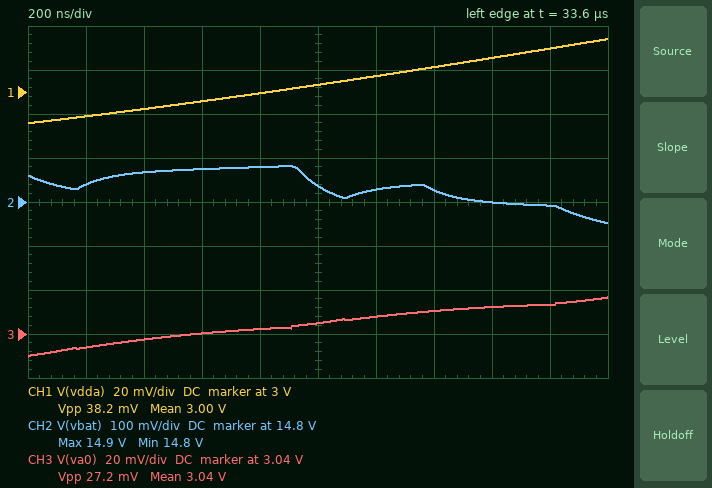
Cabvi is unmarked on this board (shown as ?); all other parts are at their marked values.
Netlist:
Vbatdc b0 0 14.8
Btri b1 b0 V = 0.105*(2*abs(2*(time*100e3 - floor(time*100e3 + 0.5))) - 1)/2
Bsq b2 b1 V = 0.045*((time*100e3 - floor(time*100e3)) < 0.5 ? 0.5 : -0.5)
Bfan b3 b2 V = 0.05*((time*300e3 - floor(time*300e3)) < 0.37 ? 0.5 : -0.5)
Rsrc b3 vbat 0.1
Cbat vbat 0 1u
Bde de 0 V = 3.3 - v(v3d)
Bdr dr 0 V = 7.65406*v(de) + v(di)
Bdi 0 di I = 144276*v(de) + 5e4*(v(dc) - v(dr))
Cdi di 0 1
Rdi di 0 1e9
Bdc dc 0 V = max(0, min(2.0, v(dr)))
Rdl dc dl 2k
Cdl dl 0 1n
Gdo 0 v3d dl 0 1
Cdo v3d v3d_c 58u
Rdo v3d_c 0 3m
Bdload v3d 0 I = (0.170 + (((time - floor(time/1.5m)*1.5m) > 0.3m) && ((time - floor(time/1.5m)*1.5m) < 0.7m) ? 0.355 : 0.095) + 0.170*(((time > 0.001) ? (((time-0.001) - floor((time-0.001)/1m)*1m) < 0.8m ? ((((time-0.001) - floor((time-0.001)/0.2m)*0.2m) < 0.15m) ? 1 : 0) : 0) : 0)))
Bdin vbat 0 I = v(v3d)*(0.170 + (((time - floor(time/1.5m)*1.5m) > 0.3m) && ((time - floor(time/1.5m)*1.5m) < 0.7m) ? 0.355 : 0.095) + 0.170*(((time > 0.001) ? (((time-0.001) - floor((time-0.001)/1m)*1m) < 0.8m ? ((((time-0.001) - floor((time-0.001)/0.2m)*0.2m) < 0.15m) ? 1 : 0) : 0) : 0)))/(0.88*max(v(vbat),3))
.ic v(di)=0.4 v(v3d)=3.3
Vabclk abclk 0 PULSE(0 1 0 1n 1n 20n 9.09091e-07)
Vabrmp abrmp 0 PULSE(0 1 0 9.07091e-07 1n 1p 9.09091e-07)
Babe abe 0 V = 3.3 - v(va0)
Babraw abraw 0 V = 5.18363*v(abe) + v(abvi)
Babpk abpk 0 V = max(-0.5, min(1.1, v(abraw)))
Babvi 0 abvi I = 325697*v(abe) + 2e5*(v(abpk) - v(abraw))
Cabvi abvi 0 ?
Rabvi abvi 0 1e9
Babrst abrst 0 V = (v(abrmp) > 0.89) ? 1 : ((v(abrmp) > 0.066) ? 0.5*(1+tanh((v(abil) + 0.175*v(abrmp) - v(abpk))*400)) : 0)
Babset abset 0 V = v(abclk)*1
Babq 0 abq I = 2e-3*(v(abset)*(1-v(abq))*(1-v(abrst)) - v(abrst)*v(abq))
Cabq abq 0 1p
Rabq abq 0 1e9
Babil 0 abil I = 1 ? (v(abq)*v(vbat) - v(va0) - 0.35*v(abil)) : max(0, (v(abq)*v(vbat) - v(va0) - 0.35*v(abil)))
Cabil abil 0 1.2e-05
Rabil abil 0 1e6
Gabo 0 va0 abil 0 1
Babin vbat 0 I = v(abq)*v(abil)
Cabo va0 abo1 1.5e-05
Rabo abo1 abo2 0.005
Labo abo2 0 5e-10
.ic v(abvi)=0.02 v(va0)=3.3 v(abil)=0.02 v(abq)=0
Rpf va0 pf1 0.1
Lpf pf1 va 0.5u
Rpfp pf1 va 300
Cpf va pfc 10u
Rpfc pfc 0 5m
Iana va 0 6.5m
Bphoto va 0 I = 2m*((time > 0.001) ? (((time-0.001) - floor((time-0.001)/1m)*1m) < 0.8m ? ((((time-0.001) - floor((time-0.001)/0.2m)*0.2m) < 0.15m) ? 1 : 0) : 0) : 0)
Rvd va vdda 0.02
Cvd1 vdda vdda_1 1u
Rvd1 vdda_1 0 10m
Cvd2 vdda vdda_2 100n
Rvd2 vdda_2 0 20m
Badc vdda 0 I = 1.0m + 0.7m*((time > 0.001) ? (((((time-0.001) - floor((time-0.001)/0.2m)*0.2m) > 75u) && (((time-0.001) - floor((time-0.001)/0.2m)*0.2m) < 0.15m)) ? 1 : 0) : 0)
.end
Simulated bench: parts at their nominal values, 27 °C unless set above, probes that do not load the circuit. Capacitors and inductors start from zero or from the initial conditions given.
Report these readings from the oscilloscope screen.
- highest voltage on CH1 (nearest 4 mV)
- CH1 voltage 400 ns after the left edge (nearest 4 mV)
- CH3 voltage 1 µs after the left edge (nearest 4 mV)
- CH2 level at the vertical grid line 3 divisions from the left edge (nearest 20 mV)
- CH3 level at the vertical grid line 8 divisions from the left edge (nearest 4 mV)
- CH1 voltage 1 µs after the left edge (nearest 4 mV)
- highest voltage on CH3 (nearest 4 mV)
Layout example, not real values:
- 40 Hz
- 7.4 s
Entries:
- 3.024 V
- 2.992 V
- 3.044 V
- 14.88 V
- 3.052 V
- 3.004 V
- 3.056 V
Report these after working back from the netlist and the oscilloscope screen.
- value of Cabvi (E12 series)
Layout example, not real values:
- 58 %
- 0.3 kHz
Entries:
- 1.5 F
